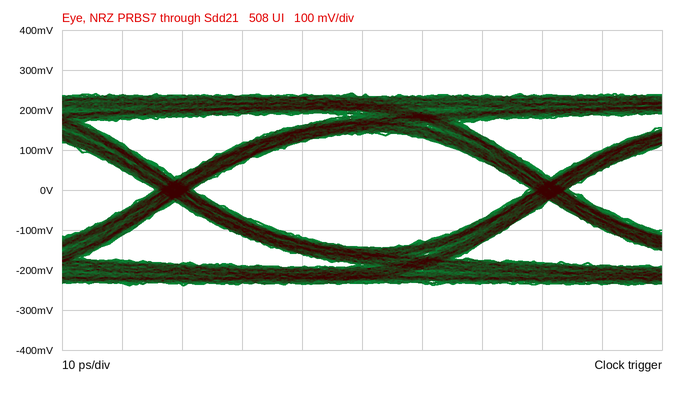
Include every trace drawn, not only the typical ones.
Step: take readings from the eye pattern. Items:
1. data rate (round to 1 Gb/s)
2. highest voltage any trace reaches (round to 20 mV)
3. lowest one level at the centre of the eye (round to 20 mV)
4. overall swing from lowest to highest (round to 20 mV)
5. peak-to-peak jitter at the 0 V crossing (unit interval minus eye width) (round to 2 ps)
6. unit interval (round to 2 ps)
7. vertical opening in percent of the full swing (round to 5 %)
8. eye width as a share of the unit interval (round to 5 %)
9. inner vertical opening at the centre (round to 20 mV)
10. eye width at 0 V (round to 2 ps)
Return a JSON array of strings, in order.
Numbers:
["16 Gb/s", "240 mV", "140 mV", "480 mV", "6 ps", "62 ps", "60 %", "90 %", "280 mV", "56 ps"]
